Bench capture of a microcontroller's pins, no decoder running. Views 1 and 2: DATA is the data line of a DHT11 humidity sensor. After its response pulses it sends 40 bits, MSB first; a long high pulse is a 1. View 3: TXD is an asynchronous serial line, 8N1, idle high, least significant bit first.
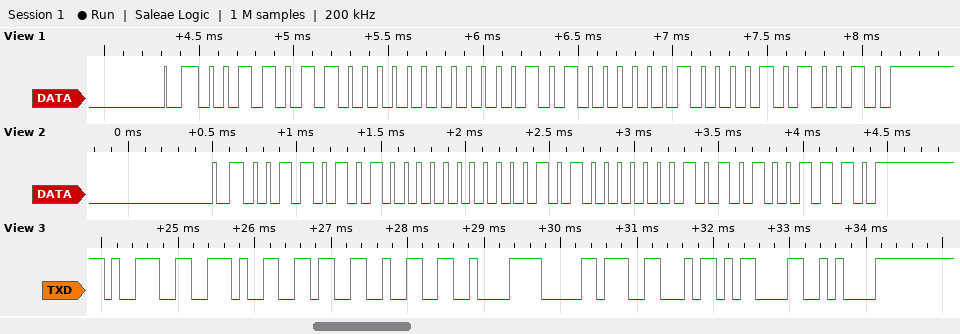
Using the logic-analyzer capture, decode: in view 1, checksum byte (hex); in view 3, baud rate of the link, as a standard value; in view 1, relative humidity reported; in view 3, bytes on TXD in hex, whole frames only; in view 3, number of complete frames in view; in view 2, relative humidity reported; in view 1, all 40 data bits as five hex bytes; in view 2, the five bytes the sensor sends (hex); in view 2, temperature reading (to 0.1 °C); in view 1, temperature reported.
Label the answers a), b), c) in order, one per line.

a) 0x52
b) 9600 baud
c) 54 %
d) 39 2E 36 32 C2 B0 46 0D 0A
e) 9
f) 53 %
g) 36 00 14 08 52
h) 35 00 14 05 4E
i) 20.5 °C
j) 20.8 °C
